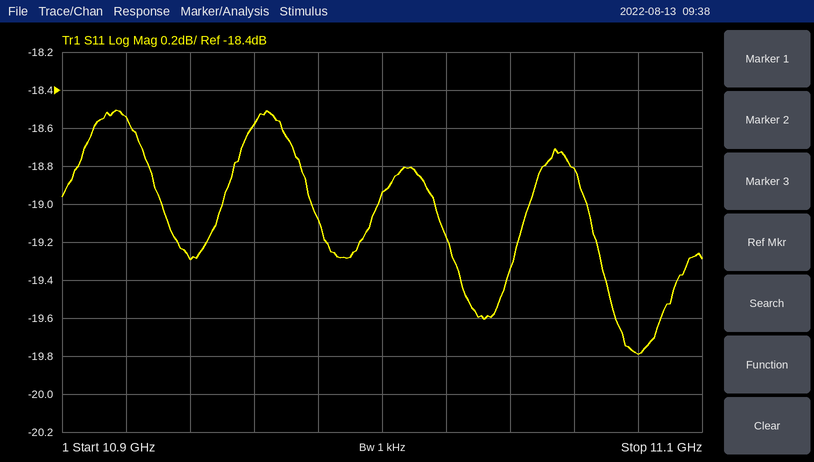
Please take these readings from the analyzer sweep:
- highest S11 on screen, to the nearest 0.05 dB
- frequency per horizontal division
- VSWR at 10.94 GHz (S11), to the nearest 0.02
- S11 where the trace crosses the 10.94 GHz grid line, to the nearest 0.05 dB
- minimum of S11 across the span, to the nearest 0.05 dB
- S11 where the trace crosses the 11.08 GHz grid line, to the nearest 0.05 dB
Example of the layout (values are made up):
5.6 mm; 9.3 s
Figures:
-18.50 dB; 20 MHz; 1.24; -19.30 dB; -19.80 dB; -19.80 dB
